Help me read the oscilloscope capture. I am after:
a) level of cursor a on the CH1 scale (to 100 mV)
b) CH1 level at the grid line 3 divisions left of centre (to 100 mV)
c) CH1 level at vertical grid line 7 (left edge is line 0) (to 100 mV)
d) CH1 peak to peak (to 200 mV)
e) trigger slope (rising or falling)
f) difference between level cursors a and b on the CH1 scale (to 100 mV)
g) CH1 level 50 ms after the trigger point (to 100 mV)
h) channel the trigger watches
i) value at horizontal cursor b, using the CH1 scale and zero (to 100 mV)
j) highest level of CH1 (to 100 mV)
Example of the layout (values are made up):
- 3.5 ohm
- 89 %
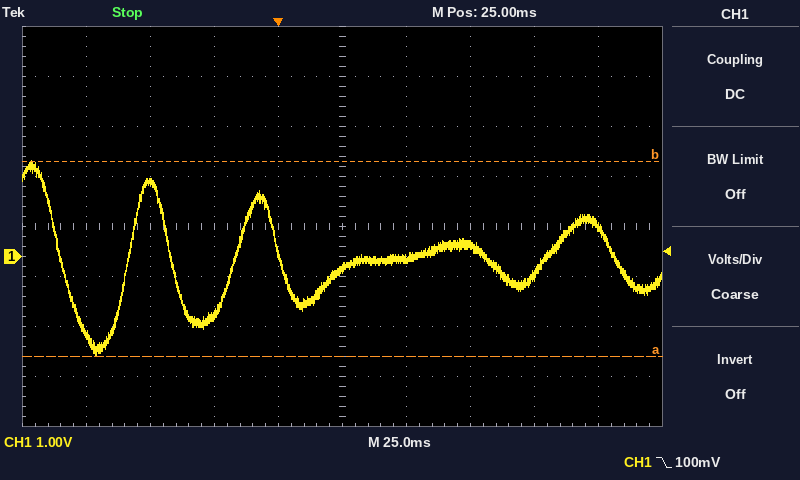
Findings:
- -2.0 V
- 1.5 V
- 200 mV
- 3.8 V
- falling
- 3.9 V
- 0.0 V
- CH1
- 1.9 V
- 1.9 V
